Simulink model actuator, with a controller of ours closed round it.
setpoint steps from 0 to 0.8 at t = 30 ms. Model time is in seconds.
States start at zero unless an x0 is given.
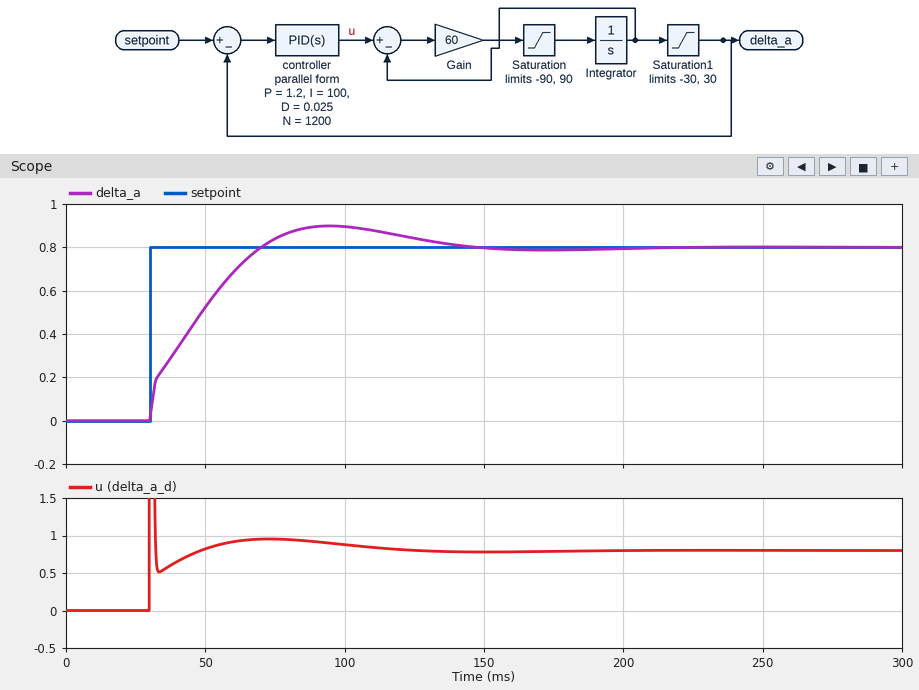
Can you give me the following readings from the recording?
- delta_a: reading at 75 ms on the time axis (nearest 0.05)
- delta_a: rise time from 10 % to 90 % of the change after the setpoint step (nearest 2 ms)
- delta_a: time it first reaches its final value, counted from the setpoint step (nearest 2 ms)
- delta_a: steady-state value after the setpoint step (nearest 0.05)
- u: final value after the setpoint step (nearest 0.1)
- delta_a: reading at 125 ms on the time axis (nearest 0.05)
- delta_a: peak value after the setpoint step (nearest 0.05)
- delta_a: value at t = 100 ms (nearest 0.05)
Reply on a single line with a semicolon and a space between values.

0.85; 32 ms; 40 ms; 0.80; 0.8; 0.85; 0.90; 0.90
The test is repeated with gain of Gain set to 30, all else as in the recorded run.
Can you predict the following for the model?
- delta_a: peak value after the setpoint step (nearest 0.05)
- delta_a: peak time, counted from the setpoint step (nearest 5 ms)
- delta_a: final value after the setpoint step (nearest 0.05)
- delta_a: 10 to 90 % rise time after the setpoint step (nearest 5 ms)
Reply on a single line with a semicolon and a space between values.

0.95; 75 ms; 0.80; 35 ms
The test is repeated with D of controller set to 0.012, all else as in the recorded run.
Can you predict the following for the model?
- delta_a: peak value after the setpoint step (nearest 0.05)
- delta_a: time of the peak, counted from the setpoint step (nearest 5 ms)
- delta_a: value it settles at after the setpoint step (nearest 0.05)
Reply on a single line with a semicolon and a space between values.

0.85; 55 ms; 0.80
